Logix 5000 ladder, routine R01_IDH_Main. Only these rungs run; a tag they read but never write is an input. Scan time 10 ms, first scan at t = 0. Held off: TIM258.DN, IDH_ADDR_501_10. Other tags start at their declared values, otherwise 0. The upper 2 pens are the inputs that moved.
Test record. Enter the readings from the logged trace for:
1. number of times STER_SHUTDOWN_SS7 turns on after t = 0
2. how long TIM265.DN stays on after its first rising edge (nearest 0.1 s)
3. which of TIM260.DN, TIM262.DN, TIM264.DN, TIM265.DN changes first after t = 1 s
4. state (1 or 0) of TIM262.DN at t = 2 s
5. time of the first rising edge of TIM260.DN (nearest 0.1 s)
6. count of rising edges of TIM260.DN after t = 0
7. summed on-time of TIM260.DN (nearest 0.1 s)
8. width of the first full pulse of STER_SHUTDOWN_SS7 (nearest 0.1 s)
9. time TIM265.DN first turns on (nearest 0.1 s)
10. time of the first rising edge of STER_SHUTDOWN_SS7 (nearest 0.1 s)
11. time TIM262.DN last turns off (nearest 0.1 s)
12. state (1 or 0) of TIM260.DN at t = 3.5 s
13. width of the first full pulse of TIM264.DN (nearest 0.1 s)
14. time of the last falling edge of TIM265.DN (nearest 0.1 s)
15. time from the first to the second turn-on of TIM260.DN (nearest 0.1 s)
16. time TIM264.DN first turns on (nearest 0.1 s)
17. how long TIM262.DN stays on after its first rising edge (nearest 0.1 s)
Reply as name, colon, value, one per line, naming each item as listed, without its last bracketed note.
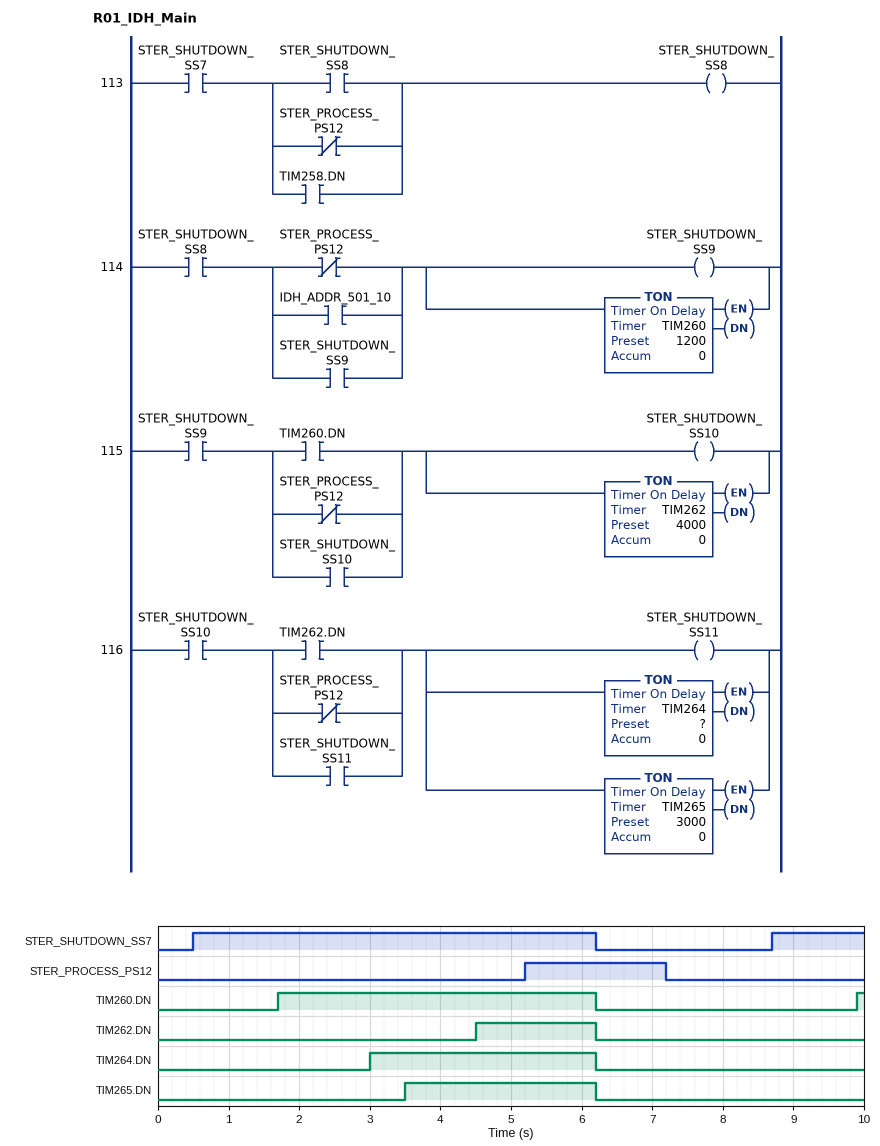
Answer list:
number of times STER_SHUTDOWN_SS7 turns on after t = 0: 2
how long TIM265.DN stays on after its first rising edge: 2.7 s
which of TIM260.DN, TIM262.DN, TIM264.DN, TIM265.DN changes first after t = 1 s: TIM260.DN
state (1 or 0) of TIM262.DN at t = 2 s: 0
time of the first rising edge of TIM260.DN: 1.7 s
count of rising edges of TIM260.DN after t = 0: 2
summed on-time of TIM260.DN: 4.6 s
width of the first full pulse of STER_SHUTDOWN_SS7: 5.7 s
time TIM265.DN first turns on: 3.5 s
time of the first rising edge of STER_SHUTDOWN_SS7: 0.5 s
time TIM262.DN last turns off: 6.2 s
state (1 or 0) of TIM260.DN at t = 3.5 s: 1
width of the first full pulse of TIM264.DN: 3.2 s
time of the last falling edge of TIM265.DN: 6.2 s
time from the first to the second turn-on of TIM260.DN: 8.2 s
time TIM264.DN first turns on: 3.0 s
how long TIM262.DN stays on after its first rising edge: 1.7 s
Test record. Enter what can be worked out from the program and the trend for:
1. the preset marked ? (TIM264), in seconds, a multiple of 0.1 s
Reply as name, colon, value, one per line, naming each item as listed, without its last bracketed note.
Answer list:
the preset marked ? (TIM264), in seconds, a multiple of 0.1 s: 2.5 s
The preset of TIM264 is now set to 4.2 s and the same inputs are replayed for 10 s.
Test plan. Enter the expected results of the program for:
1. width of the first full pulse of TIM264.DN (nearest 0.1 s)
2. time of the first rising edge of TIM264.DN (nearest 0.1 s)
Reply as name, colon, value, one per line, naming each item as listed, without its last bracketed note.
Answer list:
width of the first full pulse of TIM264.DN: 1.5 s
time of the first rising edge of TIM264.DN: 4.7 s
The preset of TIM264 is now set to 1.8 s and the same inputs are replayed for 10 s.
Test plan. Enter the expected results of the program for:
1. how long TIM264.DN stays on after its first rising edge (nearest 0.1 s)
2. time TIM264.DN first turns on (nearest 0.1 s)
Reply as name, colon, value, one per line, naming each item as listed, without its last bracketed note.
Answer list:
how long TIM264.DN stays on after its first rising edge: 3.9 s
time TIM264.DN first turns on: 2.3 s
